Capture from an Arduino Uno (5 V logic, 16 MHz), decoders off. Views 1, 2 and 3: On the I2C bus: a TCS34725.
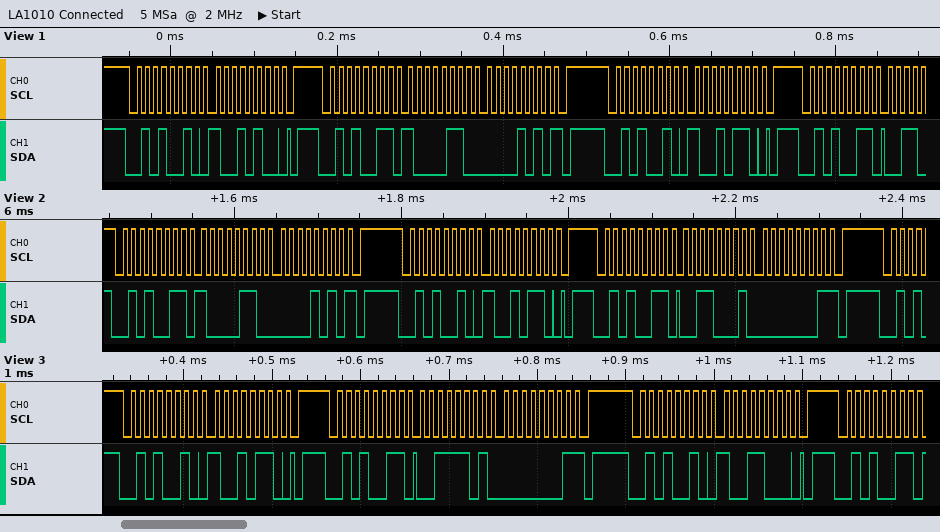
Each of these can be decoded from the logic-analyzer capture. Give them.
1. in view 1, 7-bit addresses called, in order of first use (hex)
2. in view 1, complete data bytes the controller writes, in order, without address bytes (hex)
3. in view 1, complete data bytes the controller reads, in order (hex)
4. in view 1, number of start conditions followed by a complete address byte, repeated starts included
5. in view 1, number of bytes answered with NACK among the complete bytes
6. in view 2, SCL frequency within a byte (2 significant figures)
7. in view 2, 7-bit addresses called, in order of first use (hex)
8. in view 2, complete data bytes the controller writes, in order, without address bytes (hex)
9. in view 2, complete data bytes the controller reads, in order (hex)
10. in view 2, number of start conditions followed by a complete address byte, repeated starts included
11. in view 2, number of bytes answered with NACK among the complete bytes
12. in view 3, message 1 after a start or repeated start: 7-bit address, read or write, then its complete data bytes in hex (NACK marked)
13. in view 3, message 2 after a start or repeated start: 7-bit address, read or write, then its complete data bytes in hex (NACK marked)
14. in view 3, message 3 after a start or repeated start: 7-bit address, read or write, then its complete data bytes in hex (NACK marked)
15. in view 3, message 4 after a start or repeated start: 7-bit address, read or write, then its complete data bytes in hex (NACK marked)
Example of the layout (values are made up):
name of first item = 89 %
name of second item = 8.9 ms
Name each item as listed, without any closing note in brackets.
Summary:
in view 1, 7-bit addresses called, in order of first use = 0x29
in view 1, complete data bytes the controller writes, in order, without address bytes = 94 96
in view 1, complete data bytes the controller reads, in order = 86 0A
in view 1, number of start conditions followed by a complete address byte, repeated starts included = 4
in view 1, number of bytes answered with NACK among the complete bytes = 1
in view 2, SCL frequency within a byte = 100 kHz
in view 2, 7-bit addresses called, in order of first use = 0x29
in view 2, complete data bytes the controller writes, in order, without address bytes = 96
in view 2, complete data bytes the controller reads, in order = 86 0A 31 01
in view 2, number of start conditions followed by a complete address byte, repeated starts included = 3
in view 2, number of bytes answered with NACK among the complete bytes = 2
in view 3, message 1 after a start or repeated start: 7-bit address, read or write, then its complete data bytes in hex = 0x29 write: 96
in view 3, message 2 after a start or repeated start: 7-bit address, read or write, then its complete data bytes in hex = 0x29 read: 3D 01 NACK
in view 3, message 3 after a start or repeated start: 7-bit address, read or write, then its complete data bytes in hex = 0x29 write: 98
in view 3, message 4 after a start or repeated start: 7-bit address, read or write, then its complete data bytes in hex = 0x29 read
